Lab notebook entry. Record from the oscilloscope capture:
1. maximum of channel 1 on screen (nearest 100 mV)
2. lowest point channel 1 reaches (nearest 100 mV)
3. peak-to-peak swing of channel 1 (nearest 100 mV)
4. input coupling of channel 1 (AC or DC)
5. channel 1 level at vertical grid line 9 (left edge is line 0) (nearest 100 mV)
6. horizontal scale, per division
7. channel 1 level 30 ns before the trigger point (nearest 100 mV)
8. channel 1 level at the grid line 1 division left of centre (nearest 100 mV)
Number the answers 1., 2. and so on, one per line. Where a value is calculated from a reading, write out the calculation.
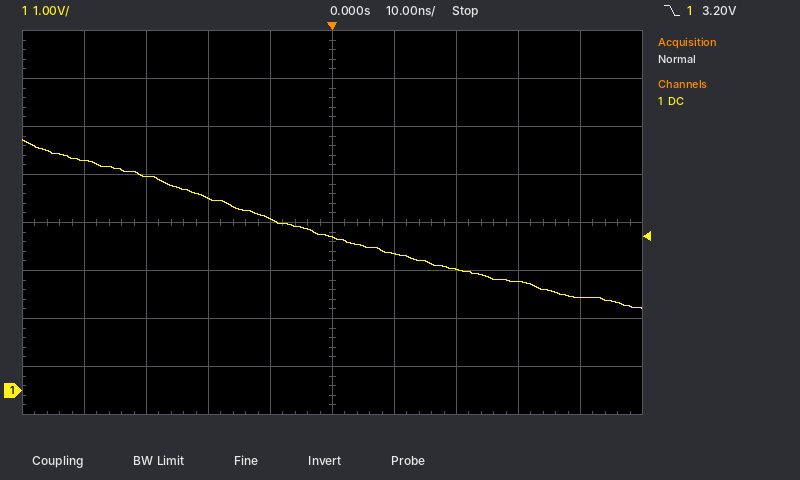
1. 5.2 V
2. 1.7 V
3. 5.2 V − (1.7 V) = 3.5 V
4. DC
5. 1.9 V
6. 10 ns
7. 4.5 V
8. 3.6 V
